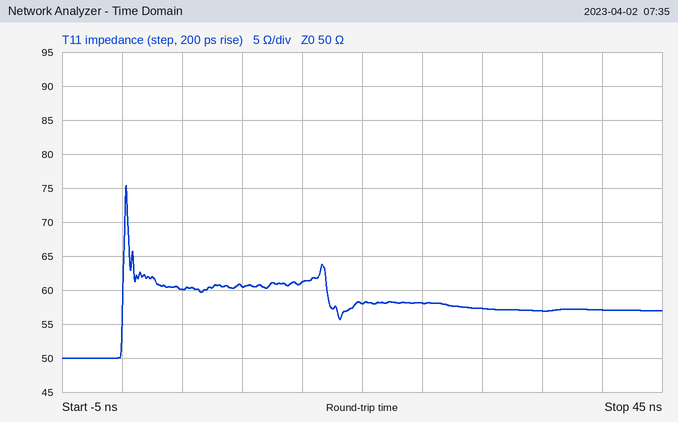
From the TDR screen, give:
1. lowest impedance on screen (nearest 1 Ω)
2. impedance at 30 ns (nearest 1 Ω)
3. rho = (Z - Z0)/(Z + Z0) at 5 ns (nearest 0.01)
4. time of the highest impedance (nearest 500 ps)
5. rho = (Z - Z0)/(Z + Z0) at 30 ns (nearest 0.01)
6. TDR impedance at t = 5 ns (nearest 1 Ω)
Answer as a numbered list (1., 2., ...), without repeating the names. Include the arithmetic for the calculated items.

1. 50 Ω
2. 57 Ω
3. (60 − 50)/(60 + 50) ≈ +0.09
4. 500 ps
5. (57 − 50)/(57 + 50) ≈ +0.07
6. 60 Ω
